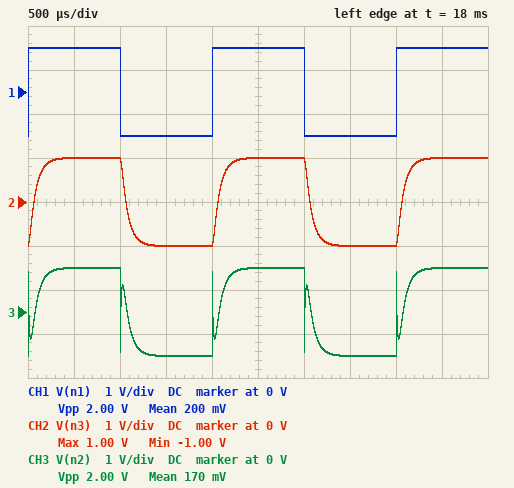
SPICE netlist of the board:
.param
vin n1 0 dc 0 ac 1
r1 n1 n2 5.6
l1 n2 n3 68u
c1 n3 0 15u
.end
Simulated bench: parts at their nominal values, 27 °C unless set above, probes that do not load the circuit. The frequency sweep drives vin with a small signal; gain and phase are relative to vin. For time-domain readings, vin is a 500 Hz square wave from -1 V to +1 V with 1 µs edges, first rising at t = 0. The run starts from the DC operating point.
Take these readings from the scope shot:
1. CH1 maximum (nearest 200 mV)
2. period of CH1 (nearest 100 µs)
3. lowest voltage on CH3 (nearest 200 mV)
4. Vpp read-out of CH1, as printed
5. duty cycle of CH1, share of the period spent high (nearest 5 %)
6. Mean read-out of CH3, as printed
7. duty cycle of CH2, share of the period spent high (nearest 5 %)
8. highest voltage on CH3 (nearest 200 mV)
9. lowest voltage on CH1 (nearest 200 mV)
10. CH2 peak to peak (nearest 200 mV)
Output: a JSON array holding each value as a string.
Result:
["1.0 V", "2.0 ms", "-1.0 V", "2.00 V", "50 %", "170 mV", "50 %", "1.0 V", "-1.0 V", "2.0 V"]
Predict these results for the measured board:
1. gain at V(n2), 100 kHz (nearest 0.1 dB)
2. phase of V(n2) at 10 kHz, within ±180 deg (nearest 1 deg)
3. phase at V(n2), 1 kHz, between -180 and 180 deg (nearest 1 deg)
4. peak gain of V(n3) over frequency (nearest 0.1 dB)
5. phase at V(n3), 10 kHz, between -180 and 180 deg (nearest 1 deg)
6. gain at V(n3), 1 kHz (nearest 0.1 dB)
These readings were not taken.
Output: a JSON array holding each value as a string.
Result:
["-0.1 dB", "60 deg", "-29 deg", "0 dB", "-120 deg", "-0.8 dB"]
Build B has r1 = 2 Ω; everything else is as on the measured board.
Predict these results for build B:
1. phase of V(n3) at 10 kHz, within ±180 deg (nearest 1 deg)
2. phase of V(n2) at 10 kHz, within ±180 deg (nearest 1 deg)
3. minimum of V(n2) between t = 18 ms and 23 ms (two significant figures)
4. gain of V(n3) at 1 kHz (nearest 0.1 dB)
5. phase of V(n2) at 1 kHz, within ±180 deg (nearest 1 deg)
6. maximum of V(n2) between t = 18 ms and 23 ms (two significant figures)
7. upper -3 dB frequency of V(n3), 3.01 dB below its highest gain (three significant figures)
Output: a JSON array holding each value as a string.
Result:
["-148 deg", "32 deg", "-1.2 V", "0.2 dB", "-11 deg", "1.2 V", "5.87 kHz"]
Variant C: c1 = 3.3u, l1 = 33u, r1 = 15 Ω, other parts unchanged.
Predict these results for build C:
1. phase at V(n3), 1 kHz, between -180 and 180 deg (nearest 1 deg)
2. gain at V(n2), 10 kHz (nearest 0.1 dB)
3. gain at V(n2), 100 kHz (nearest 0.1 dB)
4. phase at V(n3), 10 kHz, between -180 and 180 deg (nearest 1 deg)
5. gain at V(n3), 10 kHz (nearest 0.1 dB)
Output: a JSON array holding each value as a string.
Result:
["-17 deg", "-14.9 dB", "-1.9 dB", "-80 deg", "-10.0 dB"]
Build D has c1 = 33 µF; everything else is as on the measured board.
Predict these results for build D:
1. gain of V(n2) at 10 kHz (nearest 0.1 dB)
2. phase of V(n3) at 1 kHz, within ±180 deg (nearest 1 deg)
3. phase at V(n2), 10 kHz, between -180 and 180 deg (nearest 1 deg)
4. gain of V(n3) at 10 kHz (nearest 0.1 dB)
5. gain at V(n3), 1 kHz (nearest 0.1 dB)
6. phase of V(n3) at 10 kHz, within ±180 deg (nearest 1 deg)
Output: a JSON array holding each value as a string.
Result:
["-5.0 dB", "-52 deg", "56 deg", "-22.9 dB", "-3.4 dB", "-124 deg"]
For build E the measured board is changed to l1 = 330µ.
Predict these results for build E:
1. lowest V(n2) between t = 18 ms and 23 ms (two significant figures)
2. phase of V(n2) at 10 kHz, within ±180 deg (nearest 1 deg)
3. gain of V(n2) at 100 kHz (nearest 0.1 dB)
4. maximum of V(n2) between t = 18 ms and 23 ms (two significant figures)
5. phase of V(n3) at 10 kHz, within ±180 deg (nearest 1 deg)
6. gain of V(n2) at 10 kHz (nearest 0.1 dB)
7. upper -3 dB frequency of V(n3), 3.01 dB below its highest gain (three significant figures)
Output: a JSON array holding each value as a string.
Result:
["-1.1 V", "16 deg", "0 dB", "1.1 V", "-164 deg", "-0.3 dB", "2.52 kHz"]
